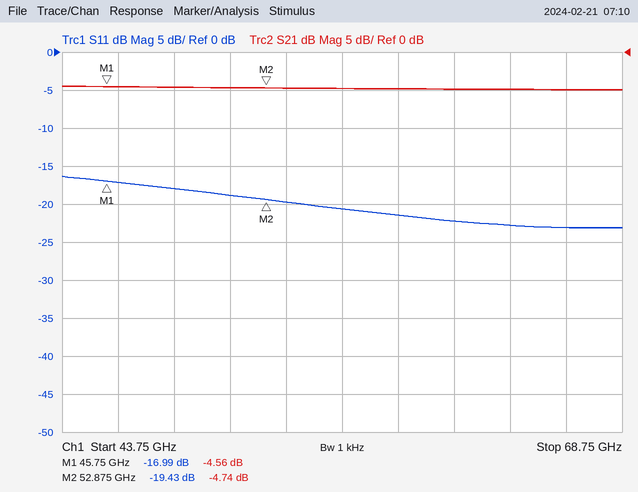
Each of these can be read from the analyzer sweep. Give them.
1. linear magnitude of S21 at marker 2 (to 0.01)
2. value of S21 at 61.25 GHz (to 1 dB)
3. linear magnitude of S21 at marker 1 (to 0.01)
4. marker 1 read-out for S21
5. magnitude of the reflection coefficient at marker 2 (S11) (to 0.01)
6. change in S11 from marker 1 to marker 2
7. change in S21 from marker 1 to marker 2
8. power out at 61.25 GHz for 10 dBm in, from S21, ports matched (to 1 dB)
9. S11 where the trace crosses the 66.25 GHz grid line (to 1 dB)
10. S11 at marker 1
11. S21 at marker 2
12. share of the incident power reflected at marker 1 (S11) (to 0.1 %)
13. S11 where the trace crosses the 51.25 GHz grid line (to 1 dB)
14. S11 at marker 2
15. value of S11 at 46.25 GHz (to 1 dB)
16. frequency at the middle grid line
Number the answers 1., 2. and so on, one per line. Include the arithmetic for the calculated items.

1. 10^(-4.74/20) ≈ 0.58
2. -5 dB
3. 10^(-4.56/20) ≈ 0.59
4. -4.56 dB
5. 10^(-19.43/20) ≈ 0.11
6. -19.43 − (-16.99) = -2.44 dB
7. -4.74 − (-4.56) = -0.18 dB
8. 10 dBm + (-5 dB) = 5 dBm
9. -23 dB
10. -16.99 dB
11. -4.74 dB
12. 10^(-16.99/10) ≈ 2.0 %
13. -19 dB
14. -19.43 dB
15. -17 dB
16. 56.25 GHz
